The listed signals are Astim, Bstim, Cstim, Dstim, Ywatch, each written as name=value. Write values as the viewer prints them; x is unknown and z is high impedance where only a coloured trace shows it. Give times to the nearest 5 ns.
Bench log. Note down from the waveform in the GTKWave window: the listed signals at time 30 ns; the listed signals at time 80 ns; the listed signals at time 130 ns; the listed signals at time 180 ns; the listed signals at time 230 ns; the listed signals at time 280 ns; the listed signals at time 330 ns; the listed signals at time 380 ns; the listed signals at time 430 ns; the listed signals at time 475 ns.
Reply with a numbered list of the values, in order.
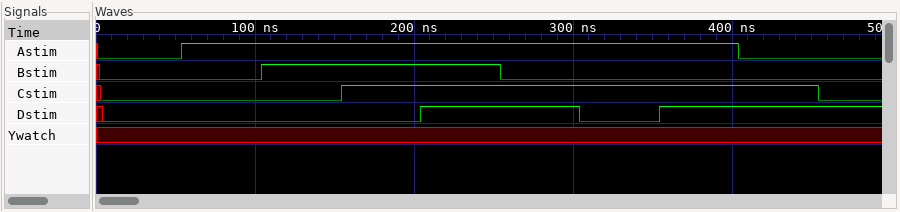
1. Astim=0, Bstim=0, Cstim=0, Dstim=0, Ywatch=x
2. Astim=1, Bstim=0, Cstim=0, Dstim=0, Ywatch=x
3. Astim=1, Bstim=1, Cstim=0, Dstim=0, Ywatch=x
4. Astim=1, Bstim=1, Cstim=1, Dstim=0, Ywatch=x
5. Astim=1, Bstim=1, Cstim=1, Dstim=1, Ywatch=x
6. Astim=1, Bstim=0, Cstim=1, Dstim=1, Ywatch=x
7. Astim=1, Bstim=0, Cstim=1, Dstim=0, Ywatch=x
8. Astim=1, Bstim=0, Cstim=1, Dstim=1, Ywatch=x
9. Astim=0, Bstim=0, Cstim=1, Dstim=1, Ywatch=x
10. Astim=0, Bstim=0, Cstim=0, Dstim=1, Ywatch=x
